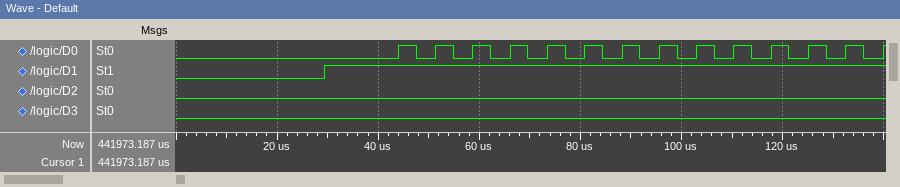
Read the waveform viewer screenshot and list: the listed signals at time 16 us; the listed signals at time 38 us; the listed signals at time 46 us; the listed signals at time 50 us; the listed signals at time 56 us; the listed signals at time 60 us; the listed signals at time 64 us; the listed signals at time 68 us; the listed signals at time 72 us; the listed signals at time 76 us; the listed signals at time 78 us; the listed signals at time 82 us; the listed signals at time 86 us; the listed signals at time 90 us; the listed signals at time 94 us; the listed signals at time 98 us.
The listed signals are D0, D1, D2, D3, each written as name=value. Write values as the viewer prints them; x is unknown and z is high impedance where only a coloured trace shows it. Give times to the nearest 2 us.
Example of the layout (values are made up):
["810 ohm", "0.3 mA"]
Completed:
["D0=0, D1=0, D2=0, D3=0", "D0=0, D1=1, D2=0, D3=0", "D0=1, D1=1, D2=0, D3=0", "D0=0, D1=1, D2=0, D3=0", "D0=0, D1=1, D2=0, D3=0", "D0=1, D1=1, D2=0, D3=0", "D0=0, D1=1, D2=0, D3=0", "D0=1, D1=1, D2=0, D3=0", "D0=0, D1=1, D2=0, D3=0", "D0=1, D1=1, D2=0, D3=0", "D0=0, D1=1, D2=0, D3=0", "D0=1, D1=1, D2=0, D3=0", "D0=0, D1=1, D2=0, D3=0", "D0=1, D1=1, D2=0, D3=0", "D0=0, D1=1, D2=0, D3=0", "D0=1, D1=1, D2=0, D3=0"]
